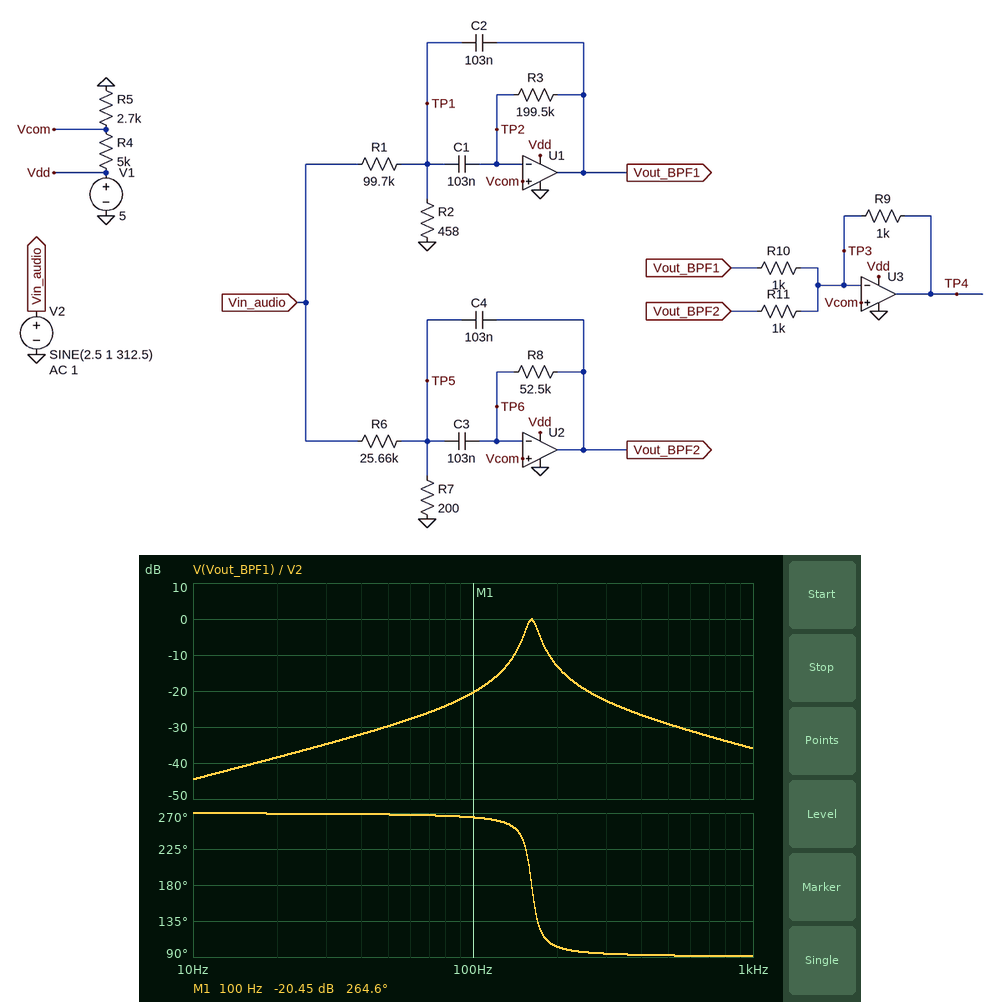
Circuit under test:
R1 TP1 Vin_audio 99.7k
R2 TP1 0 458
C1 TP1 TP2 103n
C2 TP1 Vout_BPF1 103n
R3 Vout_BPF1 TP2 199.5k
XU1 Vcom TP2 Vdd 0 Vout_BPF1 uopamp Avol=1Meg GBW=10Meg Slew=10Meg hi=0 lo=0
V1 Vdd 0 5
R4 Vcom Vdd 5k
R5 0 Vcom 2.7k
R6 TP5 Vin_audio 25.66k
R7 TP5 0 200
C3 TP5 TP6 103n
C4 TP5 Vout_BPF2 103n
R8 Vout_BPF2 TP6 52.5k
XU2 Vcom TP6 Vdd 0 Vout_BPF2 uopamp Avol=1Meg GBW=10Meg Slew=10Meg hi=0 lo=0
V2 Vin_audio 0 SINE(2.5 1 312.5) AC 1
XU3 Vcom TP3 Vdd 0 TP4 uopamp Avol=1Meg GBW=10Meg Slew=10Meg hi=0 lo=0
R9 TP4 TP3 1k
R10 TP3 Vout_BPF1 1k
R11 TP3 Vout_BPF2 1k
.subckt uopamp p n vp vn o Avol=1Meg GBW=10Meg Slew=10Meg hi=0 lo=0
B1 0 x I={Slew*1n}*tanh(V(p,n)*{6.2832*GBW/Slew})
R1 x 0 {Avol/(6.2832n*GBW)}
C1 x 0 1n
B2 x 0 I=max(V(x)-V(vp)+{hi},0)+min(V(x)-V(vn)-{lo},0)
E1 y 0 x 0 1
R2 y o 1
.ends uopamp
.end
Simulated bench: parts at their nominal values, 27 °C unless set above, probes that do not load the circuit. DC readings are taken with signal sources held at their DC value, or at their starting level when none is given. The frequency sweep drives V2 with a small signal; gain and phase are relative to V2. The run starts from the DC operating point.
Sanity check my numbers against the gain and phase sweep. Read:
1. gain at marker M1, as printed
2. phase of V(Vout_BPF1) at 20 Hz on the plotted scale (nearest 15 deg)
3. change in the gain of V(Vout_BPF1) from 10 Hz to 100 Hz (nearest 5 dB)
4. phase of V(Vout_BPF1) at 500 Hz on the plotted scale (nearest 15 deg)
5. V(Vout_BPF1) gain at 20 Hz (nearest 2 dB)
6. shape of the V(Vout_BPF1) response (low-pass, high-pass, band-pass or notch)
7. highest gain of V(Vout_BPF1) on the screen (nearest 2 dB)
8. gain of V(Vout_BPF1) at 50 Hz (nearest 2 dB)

-20.45 dB
270 deg
25 dB
90 deg
-38 dB
band-pass
0 dB
-30 dB
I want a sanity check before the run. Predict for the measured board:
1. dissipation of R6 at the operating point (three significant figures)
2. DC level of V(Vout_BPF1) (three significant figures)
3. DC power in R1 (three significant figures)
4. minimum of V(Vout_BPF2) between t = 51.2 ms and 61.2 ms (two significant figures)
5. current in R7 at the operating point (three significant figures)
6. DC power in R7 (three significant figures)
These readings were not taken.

240 µW
1.75 V
62.1 µW
1.6 V
96.7 µA
1.87 µW
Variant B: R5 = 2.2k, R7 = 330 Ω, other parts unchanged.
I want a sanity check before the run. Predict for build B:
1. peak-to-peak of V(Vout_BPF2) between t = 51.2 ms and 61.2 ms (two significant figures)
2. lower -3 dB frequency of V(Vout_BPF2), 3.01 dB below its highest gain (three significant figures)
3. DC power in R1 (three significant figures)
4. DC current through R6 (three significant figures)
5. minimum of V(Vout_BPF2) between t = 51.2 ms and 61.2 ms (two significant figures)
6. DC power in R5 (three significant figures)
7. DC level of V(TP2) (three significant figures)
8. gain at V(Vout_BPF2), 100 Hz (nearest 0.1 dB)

820 mV
345 Hz
62.1 µW
96.2 µA
1.1 V
1.06 mW
1.53 V
-26.7 dB
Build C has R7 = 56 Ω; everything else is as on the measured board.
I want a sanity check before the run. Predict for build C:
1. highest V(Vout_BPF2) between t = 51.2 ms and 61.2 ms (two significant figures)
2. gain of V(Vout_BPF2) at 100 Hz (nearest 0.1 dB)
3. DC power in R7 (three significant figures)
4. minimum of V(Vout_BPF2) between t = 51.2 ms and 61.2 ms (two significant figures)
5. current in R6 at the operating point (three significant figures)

1.8 V
-42.5 dB
529 nW
1.7 V
97.2 µA
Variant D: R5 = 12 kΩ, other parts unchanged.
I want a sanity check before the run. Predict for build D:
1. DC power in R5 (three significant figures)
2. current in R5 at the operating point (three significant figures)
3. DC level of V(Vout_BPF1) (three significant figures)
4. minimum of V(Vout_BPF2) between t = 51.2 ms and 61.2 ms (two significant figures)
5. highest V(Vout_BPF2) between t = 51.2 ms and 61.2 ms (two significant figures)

1.04 mW
294 µA
3.53 V
3.4 V
3.7 V
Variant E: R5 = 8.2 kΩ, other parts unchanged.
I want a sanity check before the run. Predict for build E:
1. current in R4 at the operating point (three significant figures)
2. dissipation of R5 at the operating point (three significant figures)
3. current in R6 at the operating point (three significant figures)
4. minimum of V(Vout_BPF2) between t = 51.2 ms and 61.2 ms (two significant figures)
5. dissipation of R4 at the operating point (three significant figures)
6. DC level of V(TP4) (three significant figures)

379 µA
1.18 mW
96.7 µA
3.0 V
717 µW
3.11 V
